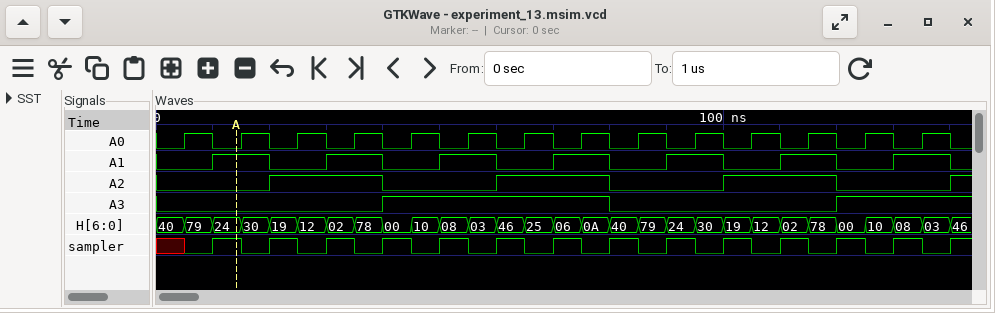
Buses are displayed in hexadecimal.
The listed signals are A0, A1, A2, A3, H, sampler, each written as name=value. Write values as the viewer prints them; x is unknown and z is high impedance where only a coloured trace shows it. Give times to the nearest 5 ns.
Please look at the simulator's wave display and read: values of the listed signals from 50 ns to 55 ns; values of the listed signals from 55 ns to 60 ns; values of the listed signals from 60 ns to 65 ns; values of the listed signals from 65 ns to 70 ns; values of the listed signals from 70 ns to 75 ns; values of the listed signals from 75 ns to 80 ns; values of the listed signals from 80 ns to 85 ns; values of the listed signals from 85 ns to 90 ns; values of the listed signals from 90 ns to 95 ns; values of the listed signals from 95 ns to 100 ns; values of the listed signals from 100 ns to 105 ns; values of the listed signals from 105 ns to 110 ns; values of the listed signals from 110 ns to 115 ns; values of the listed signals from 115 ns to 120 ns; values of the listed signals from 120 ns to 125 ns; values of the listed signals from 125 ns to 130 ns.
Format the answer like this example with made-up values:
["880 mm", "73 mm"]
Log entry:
["A0=0, A1=1, A2=0, A3=1, H=08, sampler=1", "A0=1, A1=1, A2=0, A3=1, H=03, sampler=0", "A0=0, A1=0, A2=1, A3=1, H=46, sampler=1", "A0=1, A1=0, A2=1, A3=1, H=25, sampler=0", "A0=0, A1=1, A2=1, A3=1, H=06, sampler=1", "A0=1, A1=1, A2=1, A3=1, H=0A, sampler=0", "A0=0, A1=0, A2=0, A3=0, H=40, sampler=1", "A0=1, A1=0, A2=0, A3=0, H=79, sampler=0", "A0=0, A1=1, A2=0, A3=0, H=24, sampler=1", "A0=1, A1=1, A2=0, A3=0, H=30, sampler=0", "A0=0, A1=0, A2=1, A3=0, H=19, sampler=1", "A0=1, A1=0, A2=1, A3=0, H=12, sampler=0", "A0=0, A1=1, A2=1, A3=0, H=02, sampler=1", "A0=1, A1=1, A2=1, A3=0, H=78, sampler=0", "A0=0, A1=0, A2=0, A3=1, H=00, sampler=1", "A0=1, A1=0, A2=0, A3=1, H=10, sampler=0"]
